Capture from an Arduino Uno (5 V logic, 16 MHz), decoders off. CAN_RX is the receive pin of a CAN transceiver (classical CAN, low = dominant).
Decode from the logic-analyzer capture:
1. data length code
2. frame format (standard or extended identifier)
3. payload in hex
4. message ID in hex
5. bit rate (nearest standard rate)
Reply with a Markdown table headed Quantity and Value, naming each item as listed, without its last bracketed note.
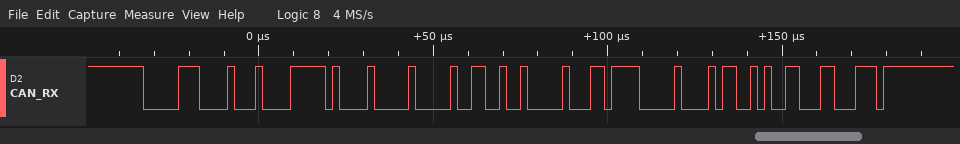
| Quantity | Value |
|---|---|
| data length code | 8 |
| frame format | standard |
| payload in hex | 7E 10 00 C9 00 DE 00 B2 |
| message ID in hex | 0x061 |
| bit rate | 500 kbit/s |
